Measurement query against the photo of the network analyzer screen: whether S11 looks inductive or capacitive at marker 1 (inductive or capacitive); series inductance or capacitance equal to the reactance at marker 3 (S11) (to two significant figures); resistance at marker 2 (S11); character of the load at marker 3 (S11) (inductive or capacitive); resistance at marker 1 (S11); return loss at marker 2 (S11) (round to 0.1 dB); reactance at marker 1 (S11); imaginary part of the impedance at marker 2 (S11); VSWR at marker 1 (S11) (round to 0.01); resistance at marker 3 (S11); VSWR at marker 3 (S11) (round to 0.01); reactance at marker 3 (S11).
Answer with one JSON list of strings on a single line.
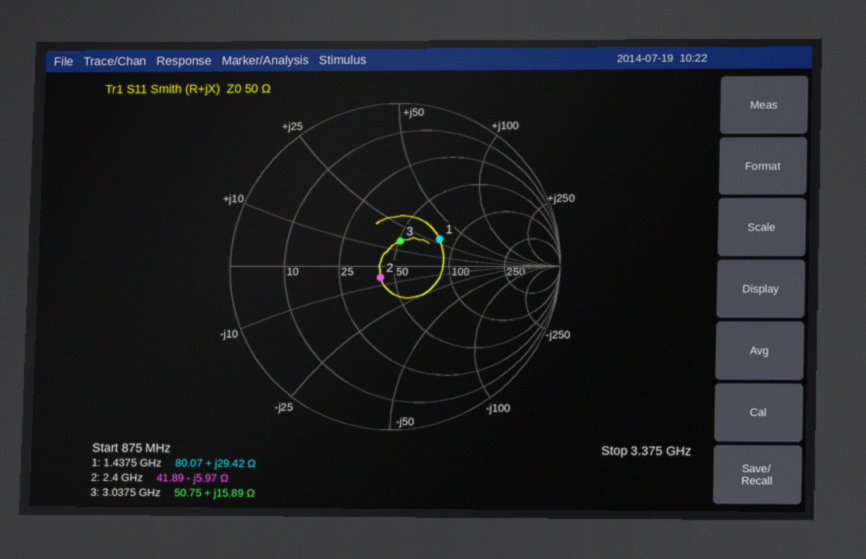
["inductive", "830 pH", "41.89 Ω", "inductive", "80.07 Ω", "19.2 dB", "+29.42 Ω", "-5.97 Ω", "1.92", "50.75 Ω", "1.37", "+15.89 Ω"]
